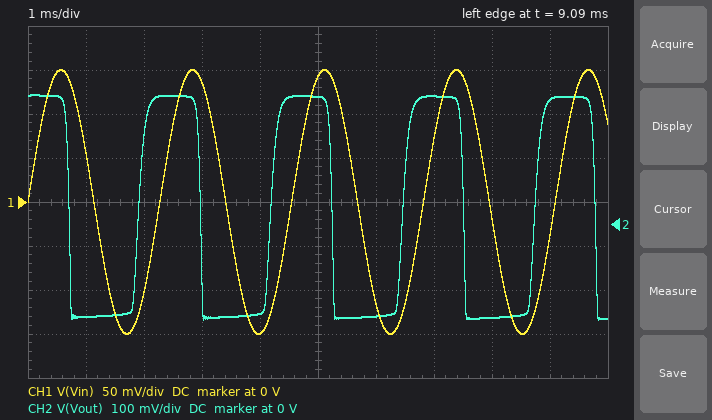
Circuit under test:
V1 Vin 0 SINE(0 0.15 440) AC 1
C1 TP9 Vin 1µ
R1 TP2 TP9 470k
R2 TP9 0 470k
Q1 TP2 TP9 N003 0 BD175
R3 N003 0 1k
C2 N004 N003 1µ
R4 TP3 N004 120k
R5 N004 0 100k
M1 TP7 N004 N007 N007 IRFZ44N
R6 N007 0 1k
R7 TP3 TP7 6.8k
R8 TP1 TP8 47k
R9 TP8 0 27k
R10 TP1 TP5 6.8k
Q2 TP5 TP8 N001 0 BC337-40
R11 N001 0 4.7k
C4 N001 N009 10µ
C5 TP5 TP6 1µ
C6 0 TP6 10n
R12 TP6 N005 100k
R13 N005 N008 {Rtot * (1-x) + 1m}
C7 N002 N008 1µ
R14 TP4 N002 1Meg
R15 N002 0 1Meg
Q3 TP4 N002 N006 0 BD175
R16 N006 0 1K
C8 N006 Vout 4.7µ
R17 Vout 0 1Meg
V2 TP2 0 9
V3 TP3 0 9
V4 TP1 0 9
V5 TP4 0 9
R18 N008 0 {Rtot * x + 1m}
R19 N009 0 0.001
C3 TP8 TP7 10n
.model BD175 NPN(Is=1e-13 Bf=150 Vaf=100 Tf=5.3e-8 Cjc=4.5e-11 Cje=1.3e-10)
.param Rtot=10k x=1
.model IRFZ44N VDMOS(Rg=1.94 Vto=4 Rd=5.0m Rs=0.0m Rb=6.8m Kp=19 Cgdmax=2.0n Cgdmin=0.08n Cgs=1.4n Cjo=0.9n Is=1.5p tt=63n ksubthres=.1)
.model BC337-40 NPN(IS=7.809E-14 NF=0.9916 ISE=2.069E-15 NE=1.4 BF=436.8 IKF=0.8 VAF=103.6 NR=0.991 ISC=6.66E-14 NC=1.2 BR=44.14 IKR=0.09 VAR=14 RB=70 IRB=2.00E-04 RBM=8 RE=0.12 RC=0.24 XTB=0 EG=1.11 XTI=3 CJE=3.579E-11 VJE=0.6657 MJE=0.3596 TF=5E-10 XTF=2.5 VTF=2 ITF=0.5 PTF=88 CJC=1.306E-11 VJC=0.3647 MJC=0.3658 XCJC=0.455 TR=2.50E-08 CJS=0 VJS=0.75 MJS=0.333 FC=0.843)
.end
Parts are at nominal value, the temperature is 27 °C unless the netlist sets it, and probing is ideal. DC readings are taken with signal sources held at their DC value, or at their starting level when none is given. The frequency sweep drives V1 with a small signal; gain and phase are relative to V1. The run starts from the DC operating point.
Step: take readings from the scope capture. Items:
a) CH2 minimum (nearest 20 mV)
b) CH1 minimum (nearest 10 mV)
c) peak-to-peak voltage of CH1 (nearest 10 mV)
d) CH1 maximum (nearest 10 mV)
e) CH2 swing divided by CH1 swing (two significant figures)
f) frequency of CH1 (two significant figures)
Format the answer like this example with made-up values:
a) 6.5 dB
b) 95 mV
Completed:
a) -220 mV
b) -150 mV
c) 300 mV
d) 150 mV
e) 1.7
f) 440 Hz
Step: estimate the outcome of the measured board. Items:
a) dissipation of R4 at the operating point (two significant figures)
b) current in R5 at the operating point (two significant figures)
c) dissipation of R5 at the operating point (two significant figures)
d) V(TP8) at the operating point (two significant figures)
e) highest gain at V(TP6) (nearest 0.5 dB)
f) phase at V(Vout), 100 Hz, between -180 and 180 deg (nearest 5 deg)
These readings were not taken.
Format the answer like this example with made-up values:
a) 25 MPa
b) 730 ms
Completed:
a) 200 µW
b) 41 µA
c) 170 µW
d) 3.3 V
e) 49.5 dB
f) 145 deg
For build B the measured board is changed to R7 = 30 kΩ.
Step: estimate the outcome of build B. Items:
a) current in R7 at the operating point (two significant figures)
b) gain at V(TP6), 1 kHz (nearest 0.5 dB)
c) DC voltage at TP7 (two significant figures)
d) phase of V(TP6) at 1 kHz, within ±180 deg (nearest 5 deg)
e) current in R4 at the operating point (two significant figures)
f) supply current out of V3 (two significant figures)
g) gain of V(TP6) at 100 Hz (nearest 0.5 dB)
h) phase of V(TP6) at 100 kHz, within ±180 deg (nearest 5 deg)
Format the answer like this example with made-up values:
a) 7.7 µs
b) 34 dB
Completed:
a) 290 µA
b) 2.0 dB
c) 290 mV
d) -15 deg
e) 41 µA
f) 330 µA
g) -27.0 dB
h) 120 deg
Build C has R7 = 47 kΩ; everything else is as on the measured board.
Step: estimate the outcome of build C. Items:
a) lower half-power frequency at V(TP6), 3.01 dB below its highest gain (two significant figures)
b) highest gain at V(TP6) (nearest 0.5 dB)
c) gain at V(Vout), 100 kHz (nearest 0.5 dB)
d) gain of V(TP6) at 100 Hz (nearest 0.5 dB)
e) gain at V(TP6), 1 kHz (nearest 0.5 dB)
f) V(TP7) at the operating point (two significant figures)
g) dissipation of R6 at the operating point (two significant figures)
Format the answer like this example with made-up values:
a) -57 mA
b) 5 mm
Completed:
a) 3.2 kHz
b) 15.5 dB
c) -13.0 dB
d) -38.5 dB
e) 1.0 dB
f) 190 mV
g) 35 µW
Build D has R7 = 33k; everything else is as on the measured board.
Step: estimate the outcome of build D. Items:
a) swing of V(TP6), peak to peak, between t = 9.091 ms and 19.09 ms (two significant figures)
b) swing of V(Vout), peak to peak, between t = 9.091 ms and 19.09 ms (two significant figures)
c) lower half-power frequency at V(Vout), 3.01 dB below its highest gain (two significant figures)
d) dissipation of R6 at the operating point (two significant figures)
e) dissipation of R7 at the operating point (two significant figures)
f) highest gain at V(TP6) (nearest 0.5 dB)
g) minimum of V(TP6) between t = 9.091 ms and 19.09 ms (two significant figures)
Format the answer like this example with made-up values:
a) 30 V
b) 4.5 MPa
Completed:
a) 5.9 V
b) 490 mV
c) 3.2 kHz
d) 70 µW
e) 2.3 mW
f) 15.5 dB
g) -2.4 V
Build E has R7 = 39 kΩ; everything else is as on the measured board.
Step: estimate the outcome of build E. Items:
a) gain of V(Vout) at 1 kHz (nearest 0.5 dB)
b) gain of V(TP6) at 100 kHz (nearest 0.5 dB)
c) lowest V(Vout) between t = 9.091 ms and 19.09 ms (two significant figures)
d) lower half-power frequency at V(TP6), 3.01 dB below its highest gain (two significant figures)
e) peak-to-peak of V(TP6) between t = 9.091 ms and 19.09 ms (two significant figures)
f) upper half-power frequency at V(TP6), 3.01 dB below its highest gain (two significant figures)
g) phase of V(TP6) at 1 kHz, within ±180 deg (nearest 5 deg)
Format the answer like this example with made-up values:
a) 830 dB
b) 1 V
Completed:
a) -20.5 dB
b) 9.0 dB
c) -6.2 mV
d) 3.2 kHz
e) 110 mV
f) 58 kHz
g) -30 deg
